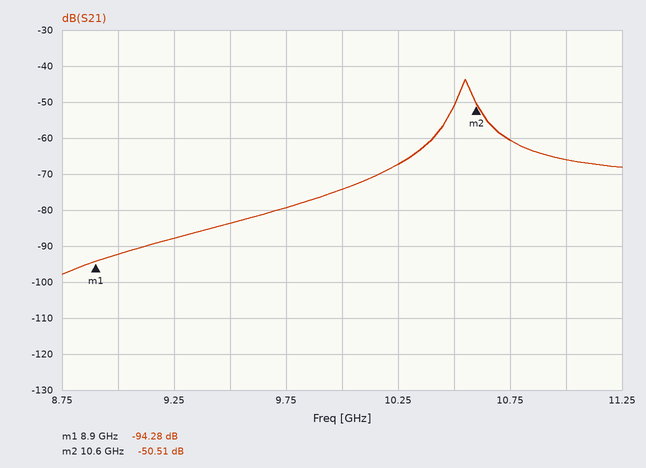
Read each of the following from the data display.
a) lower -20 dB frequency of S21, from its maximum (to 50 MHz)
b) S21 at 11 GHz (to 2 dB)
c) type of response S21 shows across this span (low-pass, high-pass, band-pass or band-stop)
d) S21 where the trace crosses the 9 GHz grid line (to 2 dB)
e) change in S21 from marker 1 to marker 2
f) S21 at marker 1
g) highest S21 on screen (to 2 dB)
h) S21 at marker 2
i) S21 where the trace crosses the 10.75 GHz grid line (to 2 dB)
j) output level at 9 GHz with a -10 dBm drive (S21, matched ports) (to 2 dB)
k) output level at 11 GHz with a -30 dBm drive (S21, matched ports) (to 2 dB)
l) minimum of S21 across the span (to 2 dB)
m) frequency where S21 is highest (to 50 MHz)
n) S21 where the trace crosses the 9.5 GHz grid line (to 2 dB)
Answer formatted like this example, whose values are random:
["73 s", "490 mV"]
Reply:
["10.35 GHz", "-66 dB", "band-pass", "-92 dB", "43.77 dB", "-94.28 dB", "-44 dB", "-50.51 dB", "-60 dB", "-102 dBm", "-96 dBm", "-98 dB", "10.55 GHz", "-84 dB"]
